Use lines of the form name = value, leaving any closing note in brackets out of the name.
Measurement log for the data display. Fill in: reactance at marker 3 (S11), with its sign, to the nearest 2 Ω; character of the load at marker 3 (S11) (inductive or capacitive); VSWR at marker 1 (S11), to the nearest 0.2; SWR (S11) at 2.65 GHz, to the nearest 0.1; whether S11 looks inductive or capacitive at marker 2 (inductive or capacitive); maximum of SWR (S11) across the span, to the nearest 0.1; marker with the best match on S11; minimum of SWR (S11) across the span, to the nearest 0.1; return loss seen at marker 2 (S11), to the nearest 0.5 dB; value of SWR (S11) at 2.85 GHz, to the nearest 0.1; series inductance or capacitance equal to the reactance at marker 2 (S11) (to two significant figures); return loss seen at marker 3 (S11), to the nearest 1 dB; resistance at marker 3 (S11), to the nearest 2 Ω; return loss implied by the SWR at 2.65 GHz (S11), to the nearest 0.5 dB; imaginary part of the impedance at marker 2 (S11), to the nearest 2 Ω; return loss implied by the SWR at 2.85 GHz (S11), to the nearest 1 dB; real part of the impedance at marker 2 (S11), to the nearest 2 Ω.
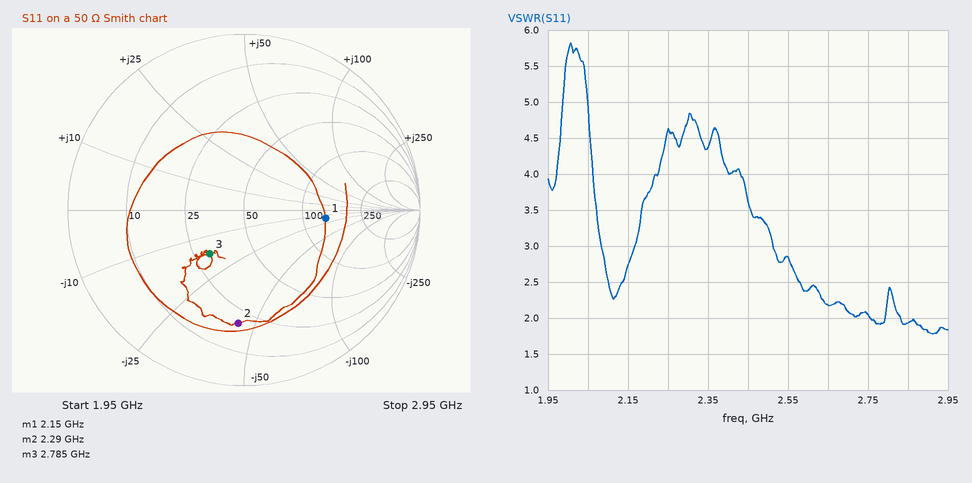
reactance at marker 3 (S11), with its sign, to the nearest 2 Ω = -16 Ω
character of the load at marker 3 (S11) = capacitive
VSWR at marker 1 (S11), to the nearest 0.2 = 2.8
SWR (S11) at 2.65 GHz, to the nearest 0.1 = 2.2
whether S11 looks inductive or capacitive at marker 2 = capacitive
maximum of SWR (S11) across the span, to the nearest 0.1 = 5.8
marker with the best match on S11 = marker 3
minimum of SWR (S11) across the span, to the nearest 0.1 = 1.8
return loss seen at marker 2 (S11), to the nearest 0.5 dB = 4.0 dB
value of SWR (S11) at 2.85 GHz, to the nearest 0.1 = 1.9
series inductance or capacitance equal to the reactance at marker 2 (S11) = 1.6 pF
return loss seen at marker 3 (S11), to the nearest 1 dB = 10 dB
resistance at marker 3 (S11), to the nearest 2 Ω = 30 Ω
return loss implied by the SWR at 2.65 GHz (S11), to the nearest 0.5 dB = 8.5 dB
imaginary part of the impedance at marker 2 (S11), to the nearest 2 Ω = -44 Ω
return loss implied by the SWR at 2.85 GHz (S11), to the nearest 1 dB = 10 dB
real part of the impedance at marker 2 (S11), to the nearest 2 Ω = 20 Ω
